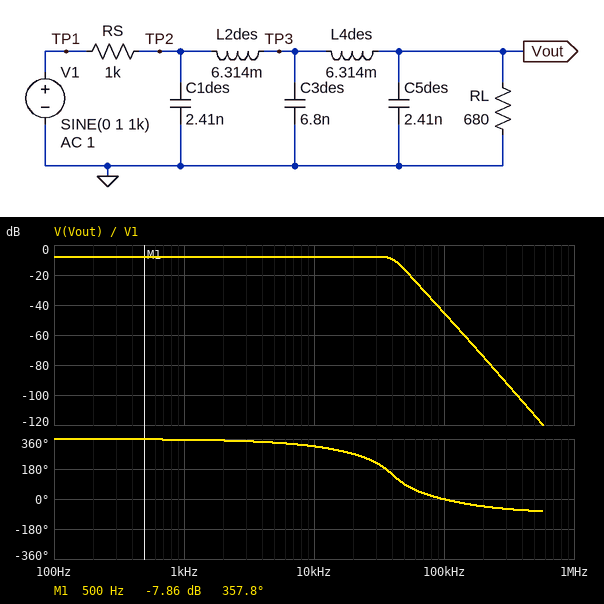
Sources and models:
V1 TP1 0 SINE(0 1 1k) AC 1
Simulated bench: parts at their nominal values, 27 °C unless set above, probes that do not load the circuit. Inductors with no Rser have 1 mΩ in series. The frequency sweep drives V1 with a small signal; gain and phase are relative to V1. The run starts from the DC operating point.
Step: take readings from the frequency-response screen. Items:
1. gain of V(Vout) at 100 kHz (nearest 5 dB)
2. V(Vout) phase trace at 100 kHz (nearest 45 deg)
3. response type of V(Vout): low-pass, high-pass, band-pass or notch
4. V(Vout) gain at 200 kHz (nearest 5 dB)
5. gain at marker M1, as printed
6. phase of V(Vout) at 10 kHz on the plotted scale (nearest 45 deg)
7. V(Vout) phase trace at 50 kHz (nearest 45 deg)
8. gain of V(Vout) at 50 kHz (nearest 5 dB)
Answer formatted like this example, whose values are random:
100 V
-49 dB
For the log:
-45 dB
0 deg
low-pass
-75 dB
-7.86 dB
315 deg
90 deg
-15 dB
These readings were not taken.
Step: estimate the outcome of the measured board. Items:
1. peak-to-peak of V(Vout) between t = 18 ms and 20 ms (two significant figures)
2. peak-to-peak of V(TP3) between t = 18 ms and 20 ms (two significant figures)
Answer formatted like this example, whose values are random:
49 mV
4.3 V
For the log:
810 mV
810 mV
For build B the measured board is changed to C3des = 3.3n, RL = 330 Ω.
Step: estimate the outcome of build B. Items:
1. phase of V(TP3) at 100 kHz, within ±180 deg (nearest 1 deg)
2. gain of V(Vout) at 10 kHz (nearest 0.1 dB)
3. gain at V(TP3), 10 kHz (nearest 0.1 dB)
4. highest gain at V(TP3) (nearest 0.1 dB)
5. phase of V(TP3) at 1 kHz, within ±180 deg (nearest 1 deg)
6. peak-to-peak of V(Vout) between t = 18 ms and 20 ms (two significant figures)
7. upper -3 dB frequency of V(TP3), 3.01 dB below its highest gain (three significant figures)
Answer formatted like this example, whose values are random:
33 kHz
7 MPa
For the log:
130 deg
-12.6 dB
-8.9 dB
4.0 dB
3 deg
500 mV
58.7 kHz
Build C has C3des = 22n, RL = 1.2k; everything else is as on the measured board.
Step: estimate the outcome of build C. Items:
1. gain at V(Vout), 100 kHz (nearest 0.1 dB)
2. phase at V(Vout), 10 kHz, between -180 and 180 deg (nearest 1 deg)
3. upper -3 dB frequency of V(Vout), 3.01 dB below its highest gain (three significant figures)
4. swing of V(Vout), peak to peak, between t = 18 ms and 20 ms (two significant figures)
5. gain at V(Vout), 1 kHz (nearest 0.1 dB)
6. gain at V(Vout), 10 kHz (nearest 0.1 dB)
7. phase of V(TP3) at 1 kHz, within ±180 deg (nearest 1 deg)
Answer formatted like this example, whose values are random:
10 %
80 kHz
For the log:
-54.1 dB
-71 deg
17.3 kHz
1.1 V
-5.3 dB
-6.4 dB
-5 deg
